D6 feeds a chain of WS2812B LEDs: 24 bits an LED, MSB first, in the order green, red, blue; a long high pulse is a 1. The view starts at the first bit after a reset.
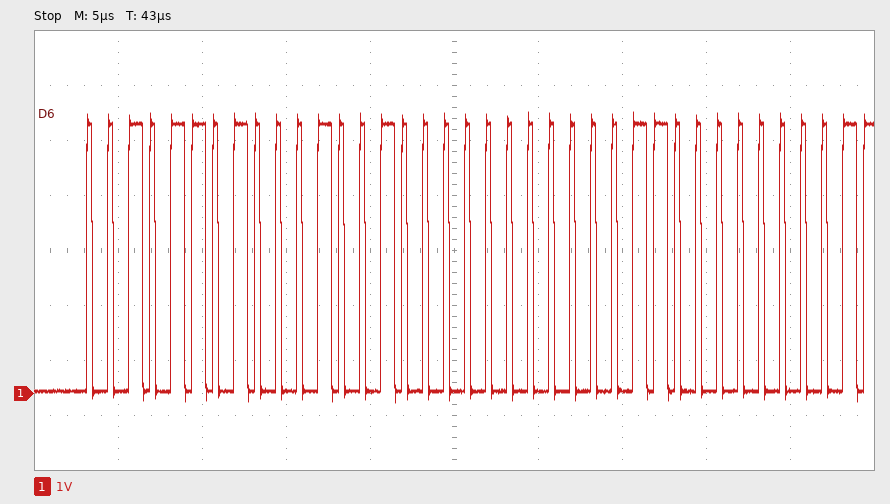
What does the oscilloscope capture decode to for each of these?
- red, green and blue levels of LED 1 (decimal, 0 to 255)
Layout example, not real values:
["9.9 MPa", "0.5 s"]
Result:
["18, 45, 0"]
